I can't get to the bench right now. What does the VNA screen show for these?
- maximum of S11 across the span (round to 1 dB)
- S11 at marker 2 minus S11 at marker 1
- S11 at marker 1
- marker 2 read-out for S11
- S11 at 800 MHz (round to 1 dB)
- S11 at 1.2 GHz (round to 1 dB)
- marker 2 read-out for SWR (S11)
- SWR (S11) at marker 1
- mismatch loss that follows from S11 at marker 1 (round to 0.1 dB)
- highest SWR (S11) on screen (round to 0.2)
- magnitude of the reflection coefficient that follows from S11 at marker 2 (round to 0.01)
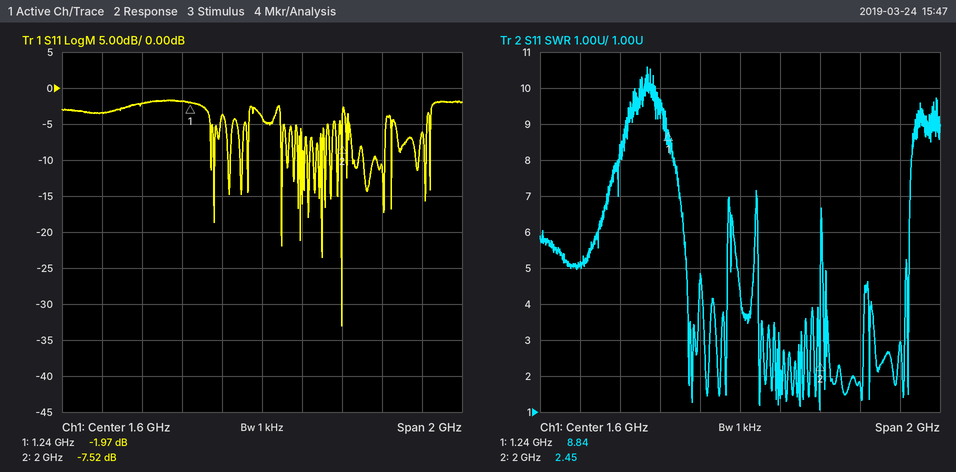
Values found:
-2 dB
-5.55 dB
-1.97 dB
-7.52 dB
-3 dB
-2 dB
2.45
8.84
4.4 dB
10.6
0.42
